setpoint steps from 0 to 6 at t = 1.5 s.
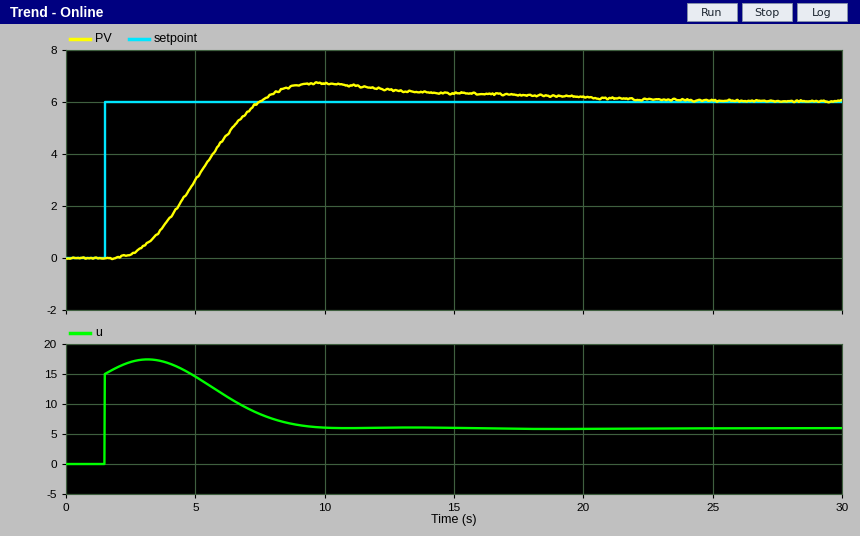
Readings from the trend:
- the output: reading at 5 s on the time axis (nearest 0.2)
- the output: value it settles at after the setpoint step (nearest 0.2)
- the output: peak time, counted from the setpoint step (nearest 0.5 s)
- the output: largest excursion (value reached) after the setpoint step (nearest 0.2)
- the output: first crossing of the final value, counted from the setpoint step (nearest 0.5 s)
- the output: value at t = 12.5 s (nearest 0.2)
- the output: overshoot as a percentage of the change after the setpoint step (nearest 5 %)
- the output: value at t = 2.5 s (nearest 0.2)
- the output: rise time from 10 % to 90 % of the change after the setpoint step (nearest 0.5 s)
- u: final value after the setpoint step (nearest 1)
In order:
3.0
6.0
8.5 s
6.8
6.0 s
6.4
10 %
0.2
3.5 s
6
